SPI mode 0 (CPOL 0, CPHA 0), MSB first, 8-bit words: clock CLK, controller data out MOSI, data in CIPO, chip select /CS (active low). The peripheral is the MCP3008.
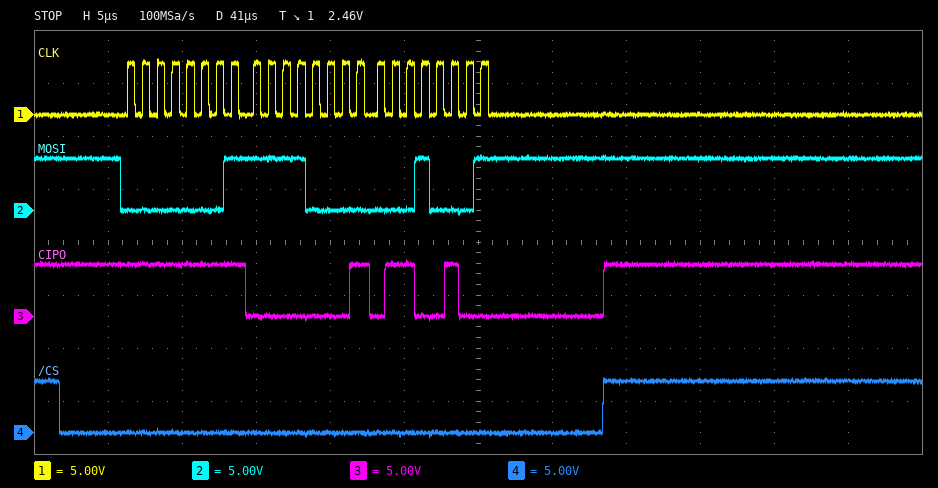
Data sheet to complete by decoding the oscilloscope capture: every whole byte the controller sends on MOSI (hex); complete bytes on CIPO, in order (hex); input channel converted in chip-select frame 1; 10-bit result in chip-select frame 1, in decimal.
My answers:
01 F0 11
FF 01 64
7
356
